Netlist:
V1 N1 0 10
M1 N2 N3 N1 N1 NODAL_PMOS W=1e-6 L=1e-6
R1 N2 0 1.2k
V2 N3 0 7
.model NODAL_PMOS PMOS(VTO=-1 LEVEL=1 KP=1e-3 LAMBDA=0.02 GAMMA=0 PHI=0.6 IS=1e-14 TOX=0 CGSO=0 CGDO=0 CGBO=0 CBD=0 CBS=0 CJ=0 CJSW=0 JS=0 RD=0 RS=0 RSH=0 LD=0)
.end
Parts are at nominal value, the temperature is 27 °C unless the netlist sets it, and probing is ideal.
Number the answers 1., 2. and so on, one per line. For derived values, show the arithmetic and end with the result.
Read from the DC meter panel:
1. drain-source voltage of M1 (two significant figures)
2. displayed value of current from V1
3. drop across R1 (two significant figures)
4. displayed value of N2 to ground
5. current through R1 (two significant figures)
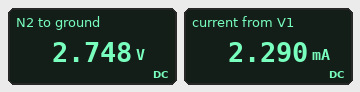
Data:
1. 2.748 V - 10 V = -7.3 V
2. 2.290 mA
3. 2.748 V = 2.7 V
4. 2.748 V
5. (2.748 V) / 1.2 kΩ = 2.3 mA
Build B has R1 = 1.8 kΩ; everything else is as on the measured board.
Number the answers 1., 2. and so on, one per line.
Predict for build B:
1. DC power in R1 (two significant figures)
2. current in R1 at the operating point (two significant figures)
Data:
1. 9.0 mW
2. 2.2 mA
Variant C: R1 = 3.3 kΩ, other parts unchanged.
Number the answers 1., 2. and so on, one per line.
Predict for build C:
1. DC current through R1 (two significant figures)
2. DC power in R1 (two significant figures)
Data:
1. 2.1 mA
2. 15 mW
